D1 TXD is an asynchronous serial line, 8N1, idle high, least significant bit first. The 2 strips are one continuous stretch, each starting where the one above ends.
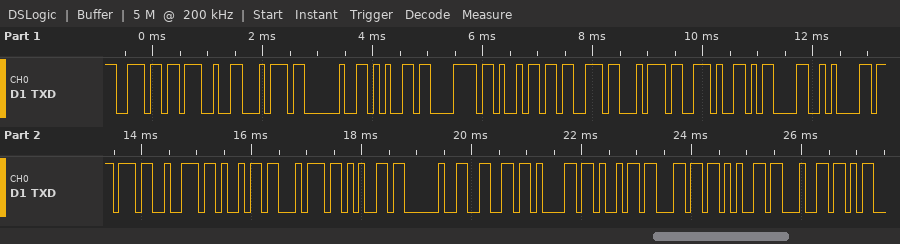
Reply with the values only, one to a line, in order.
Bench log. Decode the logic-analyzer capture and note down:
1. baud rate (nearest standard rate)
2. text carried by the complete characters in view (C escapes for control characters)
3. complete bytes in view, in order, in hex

9600 baud
"n't exist.\r\nwrite failed"
6E 27 74 20 65 78 69 73 74 2E 0D 0A 77 72 69 74 65 20 66 61 69 6C 65 64
